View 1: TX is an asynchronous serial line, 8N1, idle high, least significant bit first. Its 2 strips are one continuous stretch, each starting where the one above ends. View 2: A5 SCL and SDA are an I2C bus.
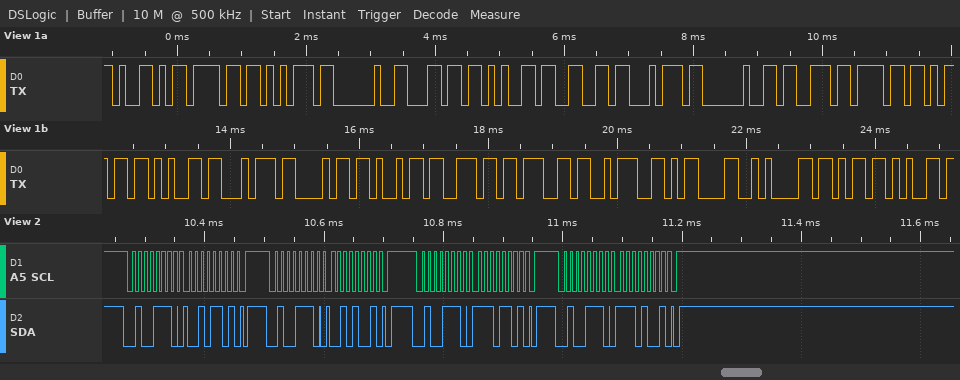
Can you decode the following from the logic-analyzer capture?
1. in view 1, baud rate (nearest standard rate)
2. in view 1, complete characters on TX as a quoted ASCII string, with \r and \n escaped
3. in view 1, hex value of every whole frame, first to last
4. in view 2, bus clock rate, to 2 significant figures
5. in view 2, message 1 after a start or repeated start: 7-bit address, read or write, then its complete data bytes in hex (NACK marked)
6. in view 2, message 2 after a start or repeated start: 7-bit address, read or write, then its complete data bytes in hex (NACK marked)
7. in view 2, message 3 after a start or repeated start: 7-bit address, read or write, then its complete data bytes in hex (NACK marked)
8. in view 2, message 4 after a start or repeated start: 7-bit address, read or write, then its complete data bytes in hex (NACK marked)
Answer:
9600 baud
"You left something:\r\nke"
0x59 0x6F 0x75 0x20 0x6C 0x65 0x66 0x74 0x20 0x73 0x6F 0x6D 0x65 0x74 0x68 0x69 0x6E 0x67 0x3A 0x0D 0x0A 0x6B 0x65
100 kHz
0x27 write: 2D
0x27 write: 29
0x27 write: ED
0x27 write: E9
